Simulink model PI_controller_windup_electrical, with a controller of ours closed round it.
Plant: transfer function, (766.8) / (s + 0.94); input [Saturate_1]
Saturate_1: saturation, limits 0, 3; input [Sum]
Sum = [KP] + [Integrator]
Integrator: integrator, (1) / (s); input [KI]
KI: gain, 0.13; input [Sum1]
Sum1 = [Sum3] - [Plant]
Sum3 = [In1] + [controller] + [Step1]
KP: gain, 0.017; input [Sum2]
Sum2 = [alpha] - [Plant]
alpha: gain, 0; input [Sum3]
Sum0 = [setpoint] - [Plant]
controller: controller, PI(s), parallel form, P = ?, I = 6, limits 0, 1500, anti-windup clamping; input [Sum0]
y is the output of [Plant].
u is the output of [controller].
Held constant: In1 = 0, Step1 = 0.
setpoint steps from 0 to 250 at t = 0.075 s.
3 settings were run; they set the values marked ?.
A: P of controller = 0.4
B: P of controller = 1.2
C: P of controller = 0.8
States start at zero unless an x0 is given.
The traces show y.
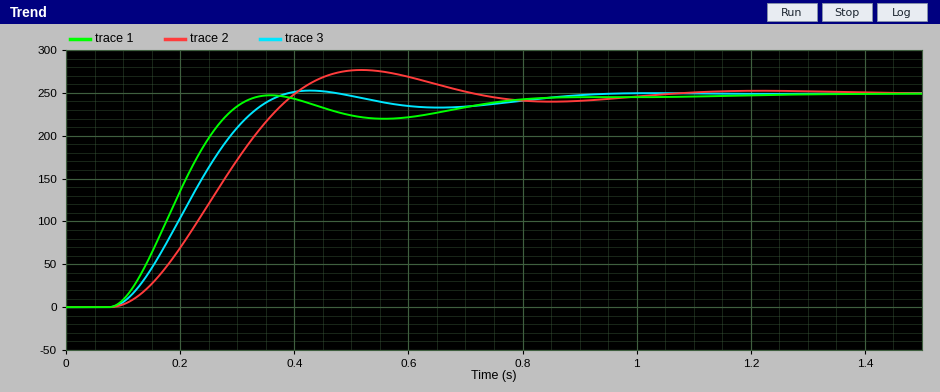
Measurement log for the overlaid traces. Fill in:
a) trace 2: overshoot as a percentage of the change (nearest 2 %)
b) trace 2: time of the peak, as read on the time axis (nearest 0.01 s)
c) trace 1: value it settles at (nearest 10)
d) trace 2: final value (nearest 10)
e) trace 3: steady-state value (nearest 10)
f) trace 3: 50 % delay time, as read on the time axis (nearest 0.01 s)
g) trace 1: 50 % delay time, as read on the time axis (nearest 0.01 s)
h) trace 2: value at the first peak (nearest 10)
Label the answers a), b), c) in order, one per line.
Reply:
a) 10 %
b) 0.52 s
c) 250
d) 250
e) 250
f) 0.22 s
g) 0.19 s
h) 280
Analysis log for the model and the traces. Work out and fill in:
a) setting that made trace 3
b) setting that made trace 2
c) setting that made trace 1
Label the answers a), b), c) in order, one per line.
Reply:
a) C
b) A
c) B
